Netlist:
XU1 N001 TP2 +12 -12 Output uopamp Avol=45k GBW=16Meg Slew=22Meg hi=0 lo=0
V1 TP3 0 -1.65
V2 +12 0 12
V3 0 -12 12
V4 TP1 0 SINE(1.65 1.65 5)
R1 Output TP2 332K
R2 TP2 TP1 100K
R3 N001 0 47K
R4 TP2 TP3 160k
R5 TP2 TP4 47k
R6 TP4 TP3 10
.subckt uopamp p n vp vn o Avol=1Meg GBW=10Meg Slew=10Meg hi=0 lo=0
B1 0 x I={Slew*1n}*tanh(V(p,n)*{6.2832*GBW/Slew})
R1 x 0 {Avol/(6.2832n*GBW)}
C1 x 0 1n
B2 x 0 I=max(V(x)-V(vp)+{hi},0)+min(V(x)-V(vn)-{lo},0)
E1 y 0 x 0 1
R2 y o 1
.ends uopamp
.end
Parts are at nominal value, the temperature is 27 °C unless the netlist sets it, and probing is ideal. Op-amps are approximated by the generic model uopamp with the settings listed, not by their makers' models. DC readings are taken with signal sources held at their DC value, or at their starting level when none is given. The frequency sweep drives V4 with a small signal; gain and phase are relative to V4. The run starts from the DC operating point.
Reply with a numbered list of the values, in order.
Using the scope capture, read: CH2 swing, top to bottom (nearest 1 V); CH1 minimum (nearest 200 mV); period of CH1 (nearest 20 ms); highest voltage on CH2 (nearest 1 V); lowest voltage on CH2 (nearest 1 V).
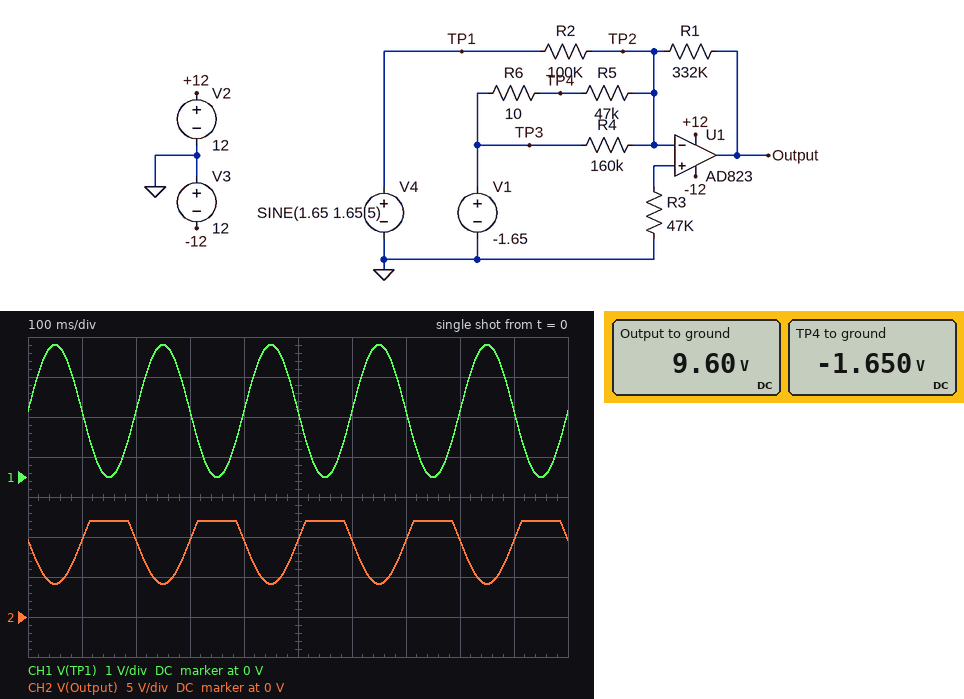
1. 8 V
2. 0 V
3. 200 ms
4. 12 V
5. 4 V
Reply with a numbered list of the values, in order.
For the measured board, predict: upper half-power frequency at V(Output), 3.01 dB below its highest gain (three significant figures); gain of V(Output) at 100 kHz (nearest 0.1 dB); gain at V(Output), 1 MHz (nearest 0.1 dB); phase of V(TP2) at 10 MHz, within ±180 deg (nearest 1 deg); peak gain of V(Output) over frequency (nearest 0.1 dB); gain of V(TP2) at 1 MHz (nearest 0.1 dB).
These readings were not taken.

1. 1.19 MHz
2. 10.4 dB
3. 8.1 dB
4. 7 deg
5. 10.4 dB
6. -16.0 dB
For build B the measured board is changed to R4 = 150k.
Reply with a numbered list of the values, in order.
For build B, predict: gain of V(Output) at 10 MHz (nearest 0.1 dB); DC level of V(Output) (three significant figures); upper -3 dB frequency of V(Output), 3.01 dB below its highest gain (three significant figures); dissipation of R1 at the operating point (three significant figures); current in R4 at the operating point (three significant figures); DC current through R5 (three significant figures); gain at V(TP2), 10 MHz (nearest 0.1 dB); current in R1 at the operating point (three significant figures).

1. -8.2 dB
2. 9.82 V
3. 1.18 MHz
4. 291 µW
5. 11.0 µA
6. 35.1 µA
7. -12.3 dB
8. 29.6 µA
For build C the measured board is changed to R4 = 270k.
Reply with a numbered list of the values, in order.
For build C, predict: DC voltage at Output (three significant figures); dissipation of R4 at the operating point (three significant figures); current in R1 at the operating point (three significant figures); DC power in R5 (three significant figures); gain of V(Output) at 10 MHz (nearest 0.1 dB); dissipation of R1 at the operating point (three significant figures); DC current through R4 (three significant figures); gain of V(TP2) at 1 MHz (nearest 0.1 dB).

1. 8.20 V
2. 10.1 µW
3. 24.7 µA
4. 57.9 µW
5. -7.6 dB
6. 203 µW
7. 6.11 µA
8. -15.8 dB
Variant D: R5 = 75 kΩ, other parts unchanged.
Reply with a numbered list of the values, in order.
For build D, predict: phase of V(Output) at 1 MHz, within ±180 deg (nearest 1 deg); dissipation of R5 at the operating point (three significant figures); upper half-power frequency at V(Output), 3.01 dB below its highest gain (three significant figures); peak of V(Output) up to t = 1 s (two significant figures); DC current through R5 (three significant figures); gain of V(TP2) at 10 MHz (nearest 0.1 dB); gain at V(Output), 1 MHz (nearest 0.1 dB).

1. 146 deg
2. 36.3 µW
3. 1.48 MHz
4. 11 V
5. 22.0 µA
6. -10.4 dB
7. 8.8 dB
